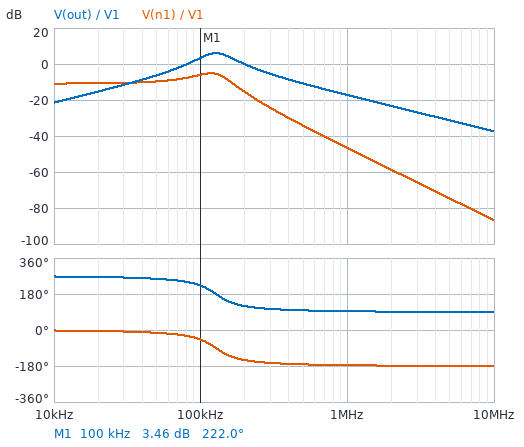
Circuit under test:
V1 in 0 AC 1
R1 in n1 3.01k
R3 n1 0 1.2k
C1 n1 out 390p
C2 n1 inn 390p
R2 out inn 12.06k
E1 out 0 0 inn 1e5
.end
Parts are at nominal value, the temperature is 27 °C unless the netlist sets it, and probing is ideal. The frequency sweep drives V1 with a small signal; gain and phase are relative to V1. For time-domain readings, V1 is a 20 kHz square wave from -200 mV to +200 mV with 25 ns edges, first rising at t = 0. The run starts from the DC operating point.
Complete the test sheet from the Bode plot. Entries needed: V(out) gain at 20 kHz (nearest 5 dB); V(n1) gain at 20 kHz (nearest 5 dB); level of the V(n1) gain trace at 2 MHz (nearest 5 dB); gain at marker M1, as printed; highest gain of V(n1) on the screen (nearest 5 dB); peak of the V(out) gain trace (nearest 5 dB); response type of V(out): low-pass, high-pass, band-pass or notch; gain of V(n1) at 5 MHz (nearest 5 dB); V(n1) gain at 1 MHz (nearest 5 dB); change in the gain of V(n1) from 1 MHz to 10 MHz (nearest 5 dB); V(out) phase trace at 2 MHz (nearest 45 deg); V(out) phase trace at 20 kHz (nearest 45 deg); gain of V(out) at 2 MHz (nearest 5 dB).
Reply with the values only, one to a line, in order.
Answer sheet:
-15 dB
-10 dB
-60 dB
3.46 dB
-5 dB
5 dB
band-pass
-75 dB
-45 dB
-40 dB
90 deg
270 deg
-25 dB
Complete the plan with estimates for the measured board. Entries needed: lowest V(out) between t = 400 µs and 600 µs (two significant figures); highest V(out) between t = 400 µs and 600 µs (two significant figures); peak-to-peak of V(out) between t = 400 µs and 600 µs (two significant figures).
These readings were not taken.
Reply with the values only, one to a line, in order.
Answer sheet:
-300 mV
300 mV
590 mV
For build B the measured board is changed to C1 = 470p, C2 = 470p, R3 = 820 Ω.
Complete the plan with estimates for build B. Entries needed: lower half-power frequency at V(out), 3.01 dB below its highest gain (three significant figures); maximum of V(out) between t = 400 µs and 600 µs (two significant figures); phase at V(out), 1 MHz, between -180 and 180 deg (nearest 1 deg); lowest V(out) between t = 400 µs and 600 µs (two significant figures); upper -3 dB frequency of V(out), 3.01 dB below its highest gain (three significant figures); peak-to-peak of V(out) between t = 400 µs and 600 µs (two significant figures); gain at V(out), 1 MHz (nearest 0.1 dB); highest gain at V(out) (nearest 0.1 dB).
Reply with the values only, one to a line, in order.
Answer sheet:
96.6 kHz
270 mV
93 deg
-270 mV
153 kHz
530 mV
-18.9 dB
6.0 dB
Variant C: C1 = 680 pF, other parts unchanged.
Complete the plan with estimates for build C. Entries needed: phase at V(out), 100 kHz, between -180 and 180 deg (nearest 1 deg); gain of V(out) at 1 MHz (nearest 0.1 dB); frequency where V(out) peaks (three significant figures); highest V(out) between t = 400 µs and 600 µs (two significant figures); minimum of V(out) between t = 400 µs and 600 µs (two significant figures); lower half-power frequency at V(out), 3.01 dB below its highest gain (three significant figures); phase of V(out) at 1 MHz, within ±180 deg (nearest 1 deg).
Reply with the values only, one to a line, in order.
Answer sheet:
172 deg
-22.1 dB
96.1 kHz
220 mV
-220 mV
73.1 kHz
93 deg
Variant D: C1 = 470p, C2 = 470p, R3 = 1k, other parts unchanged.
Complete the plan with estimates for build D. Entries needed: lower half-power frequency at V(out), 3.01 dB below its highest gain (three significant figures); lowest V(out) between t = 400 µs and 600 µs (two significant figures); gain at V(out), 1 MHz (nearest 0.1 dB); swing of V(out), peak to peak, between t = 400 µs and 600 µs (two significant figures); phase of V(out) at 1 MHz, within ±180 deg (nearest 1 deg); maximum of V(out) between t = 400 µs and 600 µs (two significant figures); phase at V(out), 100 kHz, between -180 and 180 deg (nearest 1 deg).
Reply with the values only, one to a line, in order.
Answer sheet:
87.9 kHz
-290 mV
-18.9 dB
570 mV
93 deg
290 mV
-155 deg
